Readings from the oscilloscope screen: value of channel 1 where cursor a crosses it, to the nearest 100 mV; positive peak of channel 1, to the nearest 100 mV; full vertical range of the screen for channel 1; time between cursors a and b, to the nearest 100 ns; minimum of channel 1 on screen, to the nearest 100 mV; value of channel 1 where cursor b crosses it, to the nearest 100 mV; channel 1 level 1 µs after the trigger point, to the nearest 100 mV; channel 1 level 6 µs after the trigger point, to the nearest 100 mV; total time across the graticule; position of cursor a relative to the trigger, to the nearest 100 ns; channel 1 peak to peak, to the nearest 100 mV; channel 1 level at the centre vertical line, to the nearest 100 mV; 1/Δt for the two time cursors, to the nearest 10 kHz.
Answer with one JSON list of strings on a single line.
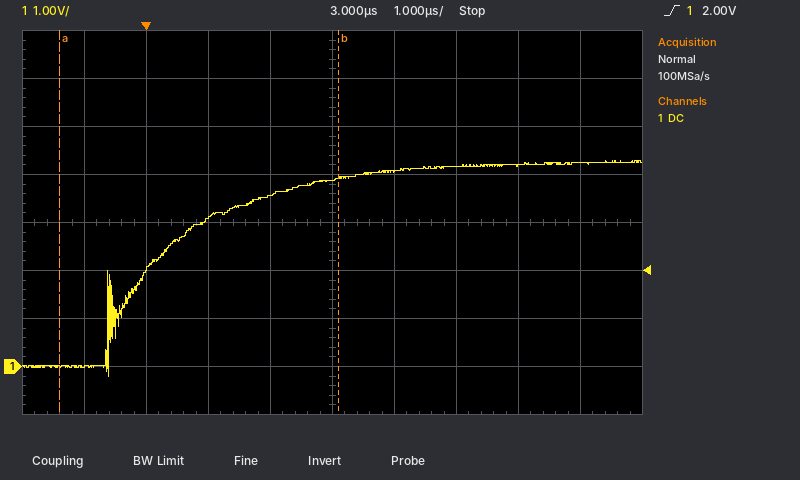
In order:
["0.0 V", "4.3 V", "8 V", "4.5 µs", "-200 mV", "3.9 V", "3.1 V", "4.2 V", "10 µs", "-1.4 µs", "4.5 V", "3.9 V", "220 kHz"]
